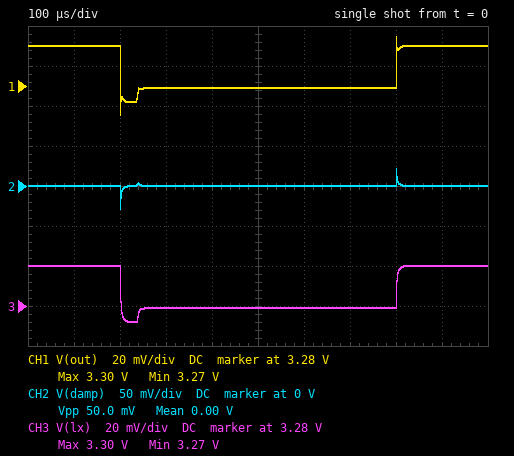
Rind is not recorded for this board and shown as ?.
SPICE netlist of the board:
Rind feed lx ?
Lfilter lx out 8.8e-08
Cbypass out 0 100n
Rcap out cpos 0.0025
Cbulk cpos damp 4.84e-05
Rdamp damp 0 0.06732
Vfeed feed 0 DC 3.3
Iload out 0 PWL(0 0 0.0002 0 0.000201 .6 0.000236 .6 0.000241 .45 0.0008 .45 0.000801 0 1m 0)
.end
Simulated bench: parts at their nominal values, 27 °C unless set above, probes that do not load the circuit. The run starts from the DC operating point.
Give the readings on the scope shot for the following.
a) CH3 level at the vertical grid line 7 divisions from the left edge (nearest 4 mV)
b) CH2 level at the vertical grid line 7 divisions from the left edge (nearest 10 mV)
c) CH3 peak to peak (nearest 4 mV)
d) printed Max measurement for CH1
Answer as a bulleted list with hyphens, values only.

- 3.280 V
- 0 V
- 28 mV
- 3.30 V
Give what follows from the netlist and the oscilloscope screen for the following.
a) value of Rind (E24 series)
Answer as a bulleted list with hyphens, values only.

- 0.047 Ω
